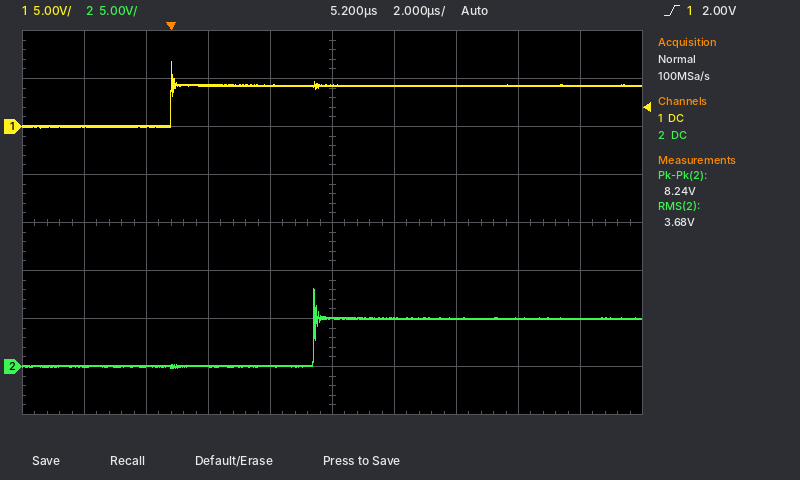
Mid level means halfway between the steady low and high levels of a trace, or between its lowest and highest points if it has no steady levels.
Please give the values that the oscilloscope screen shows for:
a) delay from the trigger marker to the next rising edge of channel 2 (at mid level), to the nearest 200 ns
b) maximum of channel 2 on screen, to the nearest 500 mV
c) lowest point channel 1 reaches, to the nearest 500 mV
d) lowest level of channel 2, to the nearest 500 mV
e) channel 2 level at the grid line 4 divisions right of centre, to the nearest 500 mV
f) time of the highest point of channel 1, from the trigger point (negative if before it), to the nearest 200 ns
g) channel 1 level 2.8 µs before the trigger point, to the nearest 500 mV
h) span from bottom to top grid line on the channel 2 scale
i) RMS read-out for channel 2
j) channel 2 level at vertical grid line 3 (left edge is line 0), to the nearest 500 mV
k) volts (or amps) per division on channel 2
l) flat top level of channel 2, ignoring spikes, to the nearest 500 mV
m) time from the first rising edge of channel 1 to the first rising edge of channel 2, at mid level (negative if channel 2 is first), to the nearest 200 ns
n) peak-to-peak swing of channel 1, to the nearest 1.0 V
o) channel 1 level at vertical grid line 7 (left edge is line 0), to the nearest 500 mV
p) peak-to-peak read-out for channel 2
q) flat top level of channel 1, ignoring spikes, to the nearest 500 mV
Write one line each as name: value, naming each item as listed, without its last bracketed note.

delay from the trigger marker to the next rising edge of channel 2 (at mid level), to the nearest 200 ns: 4.6 µs
maximum of channel 2 on screen, to the nearest 500 mV: 8.0 V
lowest point channel 1 reaches, to the nearest 500 mV: 0.0 V
lowest level of channel 2, to the nearest 500 mV: 0.0 V
channel 2 level at the grid line 4 divisions right of centre, to the nearest 500 mV: 5.0 V
time of the highest point of channel 1, from the trigger point (negative if before it), to the nearest 200 ns: 0.0 µs
channel 1 level 2.8 µs before the trigger point, to the nearest 500 mV: 0.0 V
span from bottom to top grid line on the channel 2 scale: 40 V
RMS read-out for channel 2: 3.68 V
channel 2 level at vertical grid line 3 (left edge is line 0), to the nearest 500 mV: 0.0 V
volts (or amps) per division on channel 2: 5 V
flat top level of channel 2, ignoring spikes, to the nearest 500 mV: 5.0 V
time from the first rising edge of channel 1 to the first rising edge of channel 2, at mid level (negative if channel 2 is first), to the nearest 200 ns: +4.6 µs
peak-to-peak swing of channel 1, to the nearest 1.0 V: 7.0 V
channel 1 level at vertical grid line 7 (left edge is line 0), to the nearest 500 mV: 4.5 V
peak-to-peak read-out for channel 2: 8.24 V
flat top level of channel 1, ignoring spikes, to the nearest 500 mV: 4.5 V
